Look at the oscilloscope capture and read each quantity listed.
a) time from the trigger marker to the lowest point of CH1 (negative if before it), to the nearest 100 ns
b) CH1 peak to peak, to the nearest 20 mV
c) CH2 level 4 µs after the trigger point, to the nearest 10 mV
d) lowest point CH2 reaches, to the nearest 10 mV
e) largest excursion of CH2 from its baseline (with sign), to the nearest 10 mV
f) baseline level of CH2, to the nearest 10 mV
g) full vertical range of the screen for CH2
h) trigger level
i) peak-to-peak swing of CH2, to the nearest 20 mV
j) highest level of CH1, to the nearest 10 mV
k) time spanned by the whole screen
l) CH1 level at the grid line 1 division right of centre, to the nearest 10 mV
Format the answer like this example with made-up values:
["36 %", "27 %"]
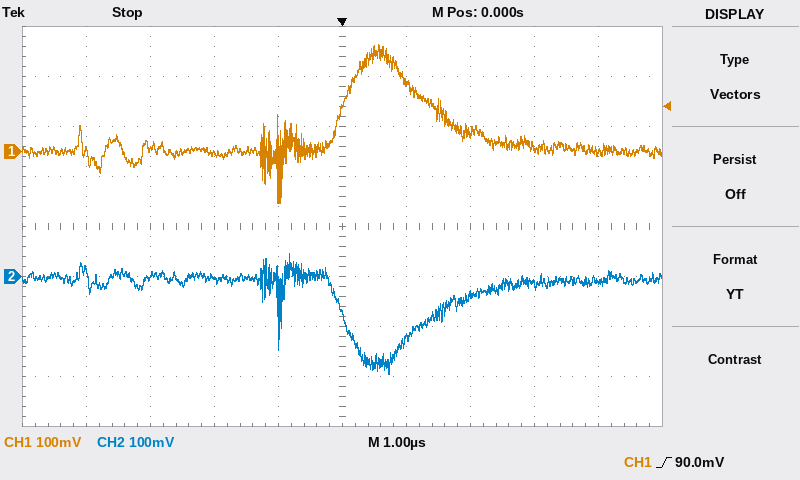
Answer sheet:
["-1.0 µs", "320 mV", "-10 mV", "-200 mV", "-190 mV", "-10 mV", "800 mV", "90.0 mV", "240 mV", "210 mV", "10 µs", "140 mV"]
